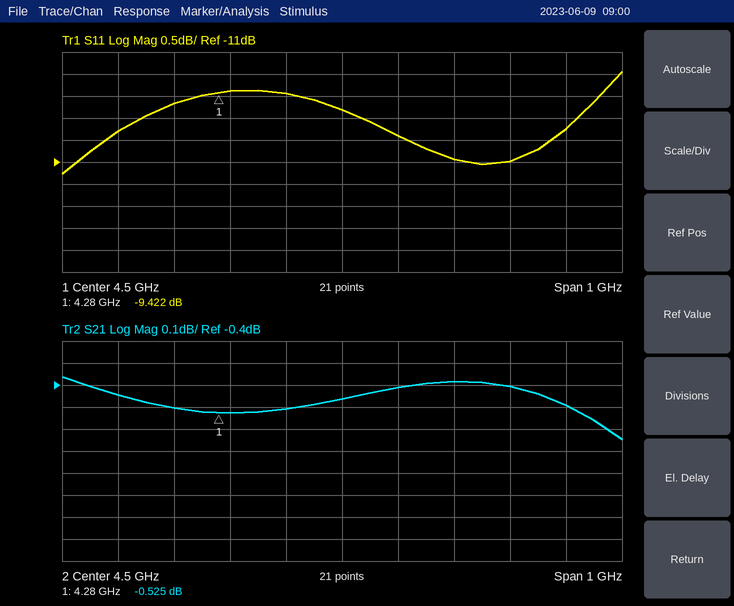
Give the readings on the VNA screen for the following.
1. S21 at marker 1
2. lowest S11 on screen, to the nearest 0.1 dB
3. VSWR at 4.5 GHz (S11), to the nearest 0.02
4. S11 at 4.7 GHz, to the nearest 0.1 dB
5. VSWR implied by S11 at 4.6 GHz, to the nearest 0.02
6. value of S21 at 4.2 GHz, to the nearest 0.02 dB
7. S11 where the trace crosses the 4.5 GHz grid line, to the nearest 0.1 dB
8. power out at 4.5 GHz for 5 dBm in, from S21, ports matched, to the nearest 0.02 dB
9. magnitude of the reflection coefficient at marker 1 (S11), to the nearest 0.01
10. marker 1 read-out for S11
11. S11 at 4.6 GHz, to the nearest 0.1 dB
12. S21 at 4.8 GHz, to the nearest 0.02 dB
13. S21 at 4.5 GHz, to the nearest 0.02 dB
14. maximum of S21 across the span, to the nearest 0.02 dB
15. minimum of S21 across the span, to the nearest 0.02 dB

-0.525 dB
-11.3 dB
1.96
-10.9 dB
1.86
-0.50 dB
-9.8 dB
4.54 dBm
0.34
-9.422 dB
-10.4 dB
-0.40 dB
-0.46 dB
-0.36 dB
-0.64 dB
